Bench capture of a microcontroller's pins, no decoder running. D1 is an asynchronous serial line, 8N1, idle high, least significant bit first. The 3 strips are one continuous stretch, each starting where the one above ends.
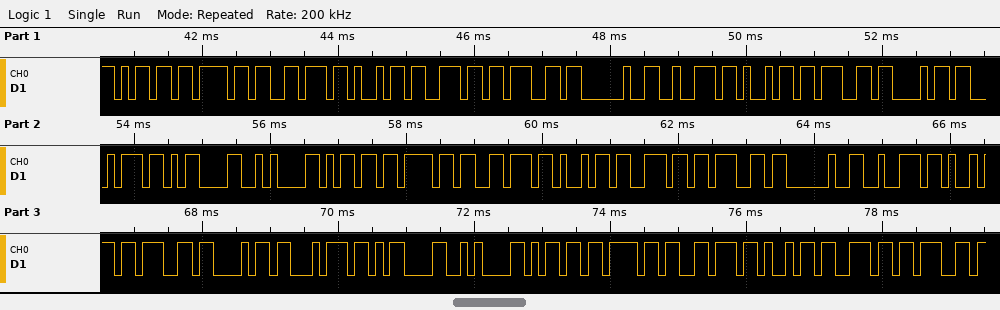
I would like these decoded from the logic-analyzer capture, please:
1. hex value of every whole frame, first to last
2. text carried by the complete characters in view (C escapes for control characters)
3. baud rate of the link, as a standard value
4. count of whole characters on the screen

6D 6F 76 69 6E 67 20 72 69 67 68 74 0D 0A 6D 6F 76 69 6E 67 20 72 69 67 68 74 0D 0A 6D 6F 76 69 6E 67
"moving right\r\nmoving right\r\nmoving"
9600 baud
34
